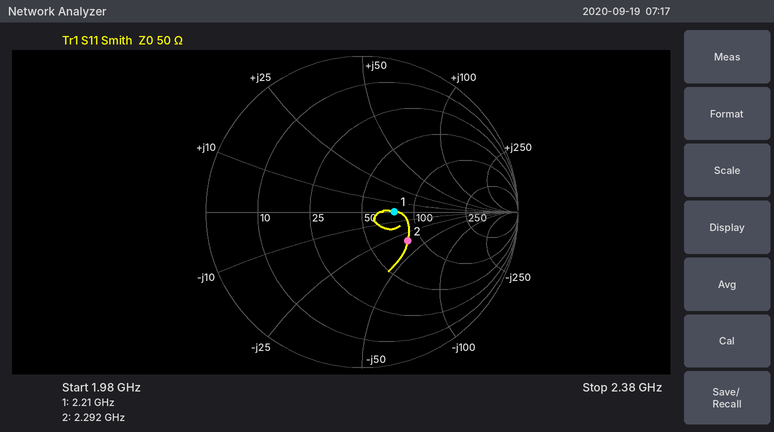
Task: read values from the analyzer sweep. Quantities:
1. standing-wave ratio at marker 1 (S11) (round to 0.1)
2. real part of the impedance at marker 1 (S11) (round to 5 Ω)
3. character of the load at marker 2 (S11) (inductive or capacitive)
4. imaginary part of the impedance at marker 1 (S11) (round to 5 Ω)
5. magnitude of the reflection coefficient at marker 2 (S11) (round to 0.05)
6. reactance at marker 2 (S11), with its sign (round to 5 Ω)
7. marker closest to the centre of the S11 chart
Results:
1.5
75 Ω
capacitive
0 Ω
0.35
-35 Ω
marker 1
